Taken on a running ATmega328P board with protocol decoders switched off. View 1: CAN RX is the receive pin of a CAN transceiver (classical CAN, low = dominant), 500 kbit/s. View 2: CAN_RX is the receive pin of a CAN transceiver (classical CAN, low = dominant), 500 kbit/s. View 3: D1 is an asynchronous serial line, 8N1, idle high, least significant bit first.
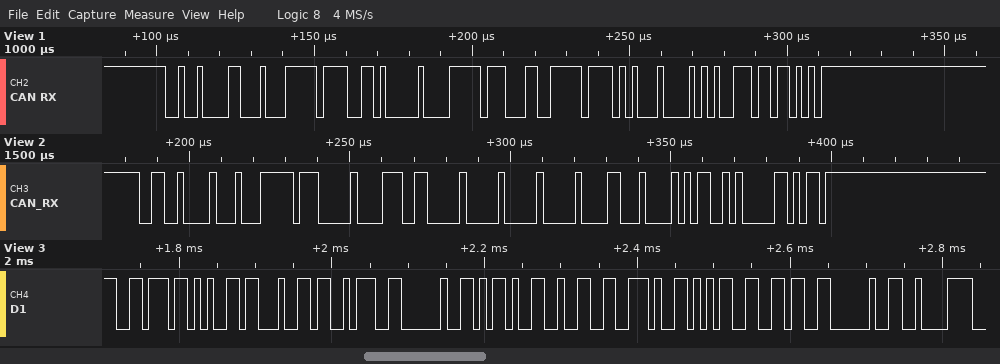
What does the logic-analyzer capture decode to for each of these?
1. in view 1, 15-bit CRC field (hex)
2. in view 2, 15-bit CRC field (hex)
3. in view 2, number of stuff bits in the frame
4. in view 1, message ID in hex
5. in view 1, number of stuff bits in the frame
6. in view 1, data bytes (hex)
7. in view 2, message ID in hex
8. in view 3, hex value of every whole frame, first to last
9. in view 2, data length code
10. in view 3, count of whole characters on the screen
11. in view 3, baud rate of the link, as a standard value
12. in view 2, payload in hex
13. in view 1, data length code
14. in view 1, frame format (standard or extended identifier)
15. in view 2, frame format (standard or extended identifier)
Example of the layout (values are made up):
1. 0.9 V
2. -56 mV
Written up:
1. 0x4EDA
2. 0x1415
3. 7
4. 0x243
5. 4
6. FF 9A 00 FF 19 FF 51 0A
7. 0x321
8. 76 65 64 3A 20 2D 32 2E 35 36 20 C2
9. 8
10. 12
11. 115200 baud
12. FF 00 73 00 00 00 C4 2B
13. 8
14. standard
15. standard
